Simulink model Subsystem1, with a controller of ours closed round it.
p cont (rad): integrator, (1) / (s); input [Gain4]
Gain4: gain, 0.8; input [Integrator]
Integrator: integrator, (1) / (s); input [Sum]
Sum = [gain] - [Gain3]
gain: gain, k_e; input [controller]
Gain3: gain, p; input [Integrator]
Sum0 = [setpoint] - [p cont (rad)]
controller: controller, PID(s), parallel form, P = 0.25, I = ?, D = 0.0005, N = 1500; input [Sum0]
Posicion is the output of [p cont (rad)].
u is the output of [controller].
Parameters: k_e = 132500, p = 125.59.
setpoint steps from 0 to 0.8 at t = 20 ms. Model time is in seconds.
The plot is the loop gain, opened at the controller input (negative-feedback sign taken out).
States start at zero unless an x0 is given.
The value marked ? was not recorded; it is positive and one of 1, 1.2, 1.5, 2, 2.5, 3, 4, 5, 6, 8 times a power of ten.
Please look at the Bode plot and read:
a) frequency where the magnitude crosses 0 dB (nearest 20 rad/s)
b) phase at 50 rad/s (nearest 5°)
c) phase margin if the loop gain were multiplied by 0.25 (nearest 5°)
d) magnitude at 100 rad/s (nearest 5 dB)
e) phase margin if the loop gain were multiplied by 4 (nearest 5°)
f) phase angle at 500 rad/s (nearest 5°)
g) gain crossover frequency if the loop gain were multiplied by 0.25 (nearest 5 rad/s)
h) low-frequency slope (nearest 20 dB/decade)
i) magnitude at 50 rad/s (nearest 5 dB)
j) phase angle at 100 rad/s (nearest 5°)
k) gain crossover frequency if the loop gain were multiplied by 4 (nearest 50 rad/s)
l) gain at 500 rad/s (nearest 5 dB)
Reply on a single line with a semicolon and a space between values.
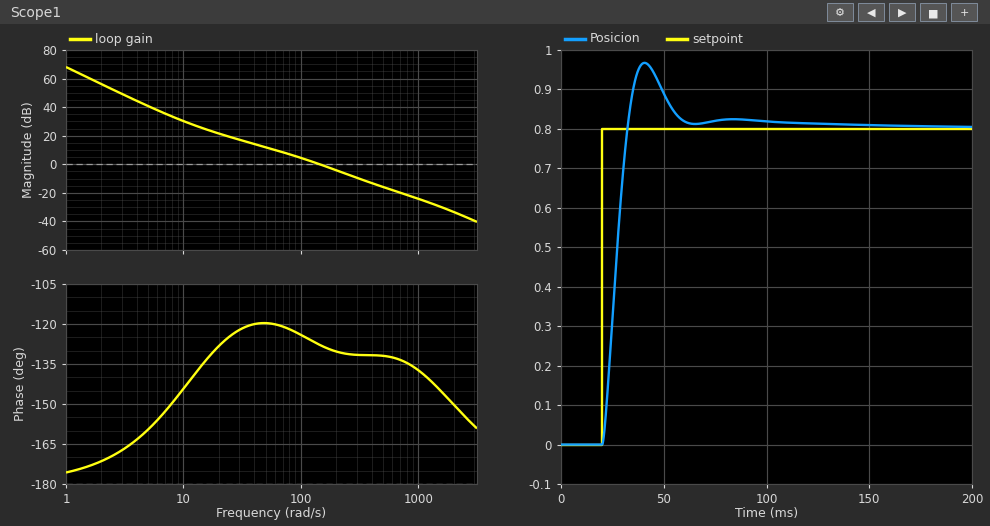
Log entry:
140 rad/s; -120°; 60°; 5 dB; 50°; -130°; 50 rad/s; -40 dB/decade; 10 dB; -125°; 350 rad/s; -15 dB
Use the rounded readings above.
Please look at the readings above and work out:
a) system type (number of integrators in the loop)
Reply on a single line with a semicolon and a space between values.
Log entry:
2
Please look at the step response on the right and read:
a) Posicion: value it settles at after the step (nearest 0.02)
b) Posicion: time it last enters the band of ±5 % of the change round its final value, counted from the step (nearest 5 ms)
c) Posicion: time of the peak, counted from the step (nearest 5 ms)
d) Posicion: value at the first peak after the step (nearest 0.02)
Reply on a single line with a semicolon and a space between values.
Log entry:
0.80; 35 ms; 20 ms; 0.96
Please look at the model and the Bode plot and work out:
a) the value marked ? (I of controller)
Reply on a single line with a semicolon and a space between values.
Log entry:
3
